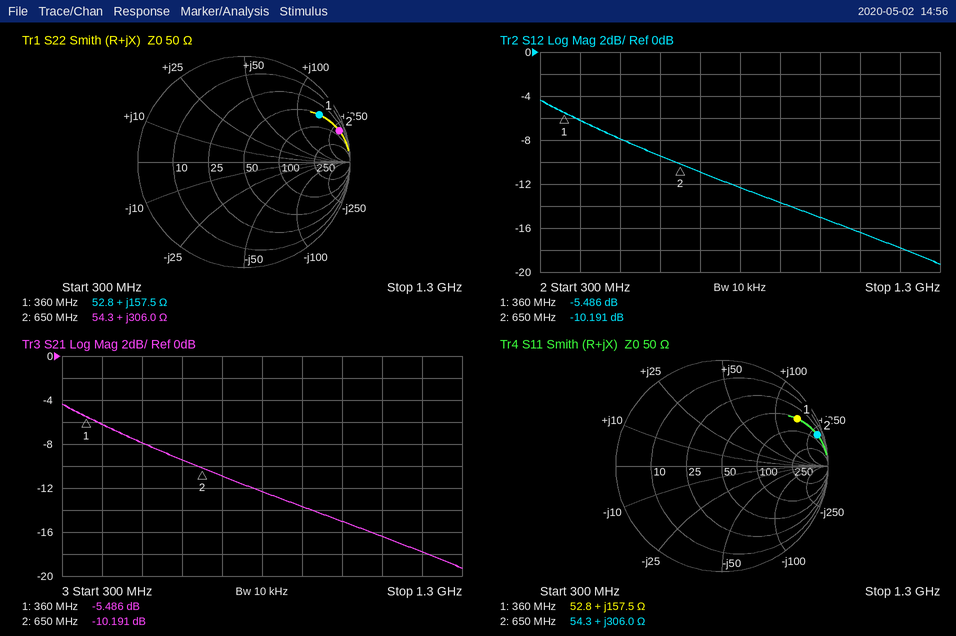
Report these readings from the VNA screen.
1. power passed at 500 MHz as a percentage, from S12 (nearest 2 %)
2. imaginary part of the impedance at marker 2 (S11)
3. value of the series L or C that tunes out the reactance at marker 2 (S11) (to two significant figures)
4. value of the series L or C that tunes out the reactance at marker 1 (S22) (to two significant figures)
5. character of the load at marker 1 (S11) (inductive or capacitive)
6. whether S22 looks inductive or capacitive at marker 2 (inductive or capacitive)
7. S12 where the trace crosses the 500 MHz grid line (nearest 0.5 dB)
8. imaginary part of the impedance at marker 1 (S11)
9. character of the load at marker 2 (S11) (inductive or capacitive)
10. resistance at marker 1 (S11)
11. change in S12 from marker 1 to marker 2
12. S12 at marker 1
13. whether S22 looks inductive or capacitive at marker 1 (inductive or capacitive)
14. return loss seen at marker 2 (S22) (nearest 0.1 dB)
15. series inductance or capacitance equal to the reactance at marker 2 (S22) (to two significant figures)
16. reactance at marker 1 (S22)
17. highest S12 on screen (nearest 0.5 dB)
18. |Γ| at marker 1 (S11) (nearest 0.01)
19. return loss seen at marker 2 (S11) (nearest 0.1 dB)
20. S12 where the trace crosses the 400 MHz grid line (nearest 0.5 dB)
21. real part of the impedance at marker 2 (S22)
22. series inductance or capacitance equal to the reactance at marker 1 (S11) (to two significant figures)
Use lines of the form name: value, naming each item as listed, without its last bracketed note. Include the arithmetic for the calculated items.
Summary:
power passed at 500 MHz as a percentage, from S12: 10^(-8/10) ≈ 16 %
imaginary part of the impedance at marker 2: +306.0 Ω
value of the series L or C that tunes out the reactance at marker 2 (S11): C = 1/(2π × 650 MHz × 306 Ω) ≈ 800 fF
value of the series L or C that tunes out the reactance at marker 1 (S22): C = 1/(2π × 360 MHz × 157.5 Ω) ≈ 2.8 pF
character of the load at marker 1 (S11): inductive
whether S22 looks inductive or capacitive at marker 2: inductive
S12 where the trace crosses the 500 MHz grid line: -8.0 dB
imaginary part of the impedance at marker 1: +157.5 Ω
character of the load at marker 2 (S11): inductive
resistance at marker 1: 52.8 Ω
change in S12 from marker 1 to marker 2: -10.191 − (-5.486) = -4.705 dB
S12 at marker 1: -5.486 dB
whether S22 looks inductive or capacitive at marker 1: inductive
return loss seen at marker 2 (S22): 0.5 dB
series inductance or capacitance equal to the reactance at marker 2 (S22): L = 306 Ω/(2π × 650 MHz) ≈ 75 nH
reactance at marker 1: +157.5 Ω
highest S12 on screen: -4.5 dB
|Γ| at marker 1 (S11): 0.84
return loss seen at marker 2 (S11): 0.5 dB
S12 where the trace crosses the 400 MHz grid line: -6.0 dB
real part of the impedance at marker 2: 54.3 Ω
series inductance or capacitance equal to the reactance at marker 1 (S11): L = 157.5 Ω/(2π × 360 MHz) ≈ 70 nH
